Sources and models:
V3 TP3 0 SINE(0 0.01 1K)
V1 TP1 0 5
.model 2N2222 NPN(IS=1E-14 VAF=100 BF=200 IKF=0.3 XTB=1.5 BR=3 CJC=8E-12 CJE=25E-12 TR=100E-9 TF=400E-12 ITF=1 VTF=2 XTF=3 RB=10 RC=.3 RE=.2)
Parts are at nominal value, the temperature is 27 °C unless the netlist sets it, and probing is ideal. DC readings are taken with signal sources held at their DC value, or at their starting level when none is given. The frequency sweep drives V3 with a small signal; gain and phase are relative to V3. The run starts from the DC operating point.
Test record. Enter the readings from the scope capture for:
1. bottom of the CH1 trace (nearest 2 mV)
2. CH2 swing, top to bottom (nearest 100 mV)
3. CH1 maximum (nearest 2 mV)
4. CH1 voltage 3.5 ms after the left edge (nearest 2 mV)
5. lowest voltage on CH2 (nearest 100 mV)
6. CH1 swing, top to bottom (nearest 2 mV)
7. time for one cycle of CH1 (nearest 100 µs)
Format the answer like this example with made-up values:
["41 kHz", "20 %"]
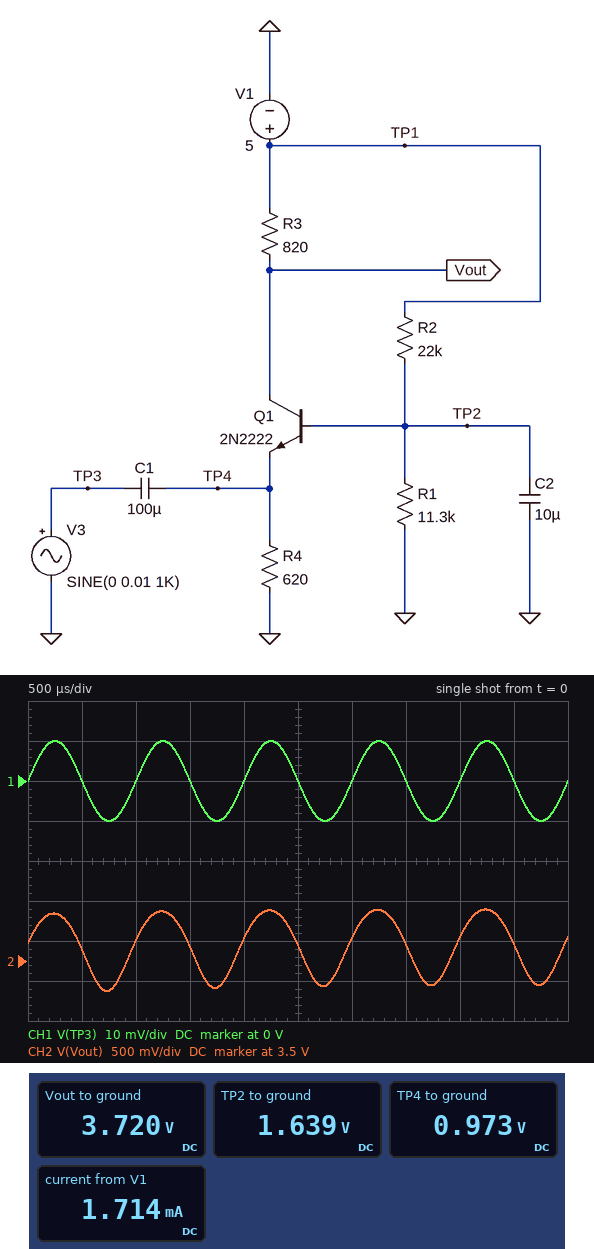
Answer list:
["-10 mV", "1.0 V", "10 mV", "0 V", "3.1 V", "20 mV", "1.0 ms"]
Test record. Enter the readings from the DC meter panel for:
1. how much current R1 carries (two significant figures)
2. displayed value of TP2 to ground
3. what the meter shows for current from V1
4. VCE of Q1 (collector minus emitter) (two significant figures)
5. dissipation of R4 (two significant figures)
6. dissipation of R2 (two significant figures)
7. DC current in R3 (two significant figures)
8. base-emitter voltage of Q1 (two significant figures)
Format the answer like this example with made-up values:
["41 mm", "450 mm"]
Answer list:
["150 µA", "1.639 V", "1.714 mA", "2.7 V", "1.5 mW", "510 µW", "1.6 mA", "670 mV"]
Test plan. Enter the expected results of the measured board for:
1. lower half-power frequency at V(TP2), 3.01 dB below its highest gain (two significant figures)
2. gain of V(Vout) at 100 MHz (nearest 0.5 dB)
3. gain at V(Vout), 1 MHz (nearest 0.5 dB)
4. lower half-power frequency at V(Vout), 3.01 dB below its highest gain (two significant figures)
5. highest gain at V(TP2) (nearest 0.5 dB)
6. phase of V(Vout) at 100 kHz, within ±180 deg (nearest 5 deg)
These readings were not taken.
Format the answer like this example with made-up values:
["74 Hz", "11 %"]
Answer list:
["2.1 Hz", "20.0 dB", "33.5 dB", "100 Hz", "-27.0 dB", "0 deg"]
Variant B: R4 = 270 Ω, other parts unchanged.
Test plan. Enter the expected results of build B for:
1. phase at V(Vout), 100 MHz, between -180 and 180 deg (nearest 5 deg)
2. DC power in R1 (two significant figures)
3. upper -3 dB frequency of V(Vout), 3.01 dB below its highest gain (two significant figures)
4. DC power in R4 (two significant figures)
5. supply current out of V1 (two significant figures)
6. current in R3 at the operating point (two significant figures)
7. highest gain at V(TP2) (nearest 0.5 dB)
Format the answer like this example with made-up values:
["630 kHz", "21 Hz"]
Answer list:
["-95 deg", "220 µW", "13 MHz", "2.9 mW", "3.4 mA", "3.3 mA", "-26.5 dB"]
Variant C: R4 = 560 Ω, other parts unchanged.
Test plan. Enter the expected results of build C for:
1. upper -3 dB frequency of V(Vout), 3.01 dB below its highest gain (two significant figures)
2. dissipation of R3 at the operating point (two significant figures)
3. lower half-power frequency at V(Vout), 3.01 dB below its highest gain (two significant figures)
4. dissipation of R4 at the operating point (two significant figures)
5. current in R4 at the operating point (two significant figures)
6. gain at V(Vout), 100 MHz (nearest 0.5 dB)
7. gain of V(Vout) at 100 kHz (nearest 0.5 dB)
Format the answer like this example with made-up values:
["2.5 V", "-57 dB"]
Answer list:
["22 MHz", "2.4 mW", "110 Hz", "1.7 mW", "1.7 mA", "20.5 dB", "34.5 dB"]
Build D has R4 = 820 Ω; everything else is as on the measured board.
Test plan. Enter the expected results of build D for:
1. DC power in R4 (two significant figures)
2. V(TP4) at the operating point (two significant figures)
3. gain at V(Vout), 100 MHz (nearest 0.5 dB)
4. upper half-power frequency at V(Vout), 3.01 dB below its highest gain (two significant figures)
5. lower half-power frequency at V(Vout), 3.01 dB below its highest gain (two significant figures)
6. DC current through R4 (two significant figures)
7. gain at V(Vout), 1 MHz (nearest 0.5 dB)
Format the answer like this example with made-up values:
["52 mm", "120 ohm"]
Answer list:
["1.2 mW", "990 mV", "19.0 dB", "26 MHz", "78 Hz", "1.2 mA", "31.5 dB"]
